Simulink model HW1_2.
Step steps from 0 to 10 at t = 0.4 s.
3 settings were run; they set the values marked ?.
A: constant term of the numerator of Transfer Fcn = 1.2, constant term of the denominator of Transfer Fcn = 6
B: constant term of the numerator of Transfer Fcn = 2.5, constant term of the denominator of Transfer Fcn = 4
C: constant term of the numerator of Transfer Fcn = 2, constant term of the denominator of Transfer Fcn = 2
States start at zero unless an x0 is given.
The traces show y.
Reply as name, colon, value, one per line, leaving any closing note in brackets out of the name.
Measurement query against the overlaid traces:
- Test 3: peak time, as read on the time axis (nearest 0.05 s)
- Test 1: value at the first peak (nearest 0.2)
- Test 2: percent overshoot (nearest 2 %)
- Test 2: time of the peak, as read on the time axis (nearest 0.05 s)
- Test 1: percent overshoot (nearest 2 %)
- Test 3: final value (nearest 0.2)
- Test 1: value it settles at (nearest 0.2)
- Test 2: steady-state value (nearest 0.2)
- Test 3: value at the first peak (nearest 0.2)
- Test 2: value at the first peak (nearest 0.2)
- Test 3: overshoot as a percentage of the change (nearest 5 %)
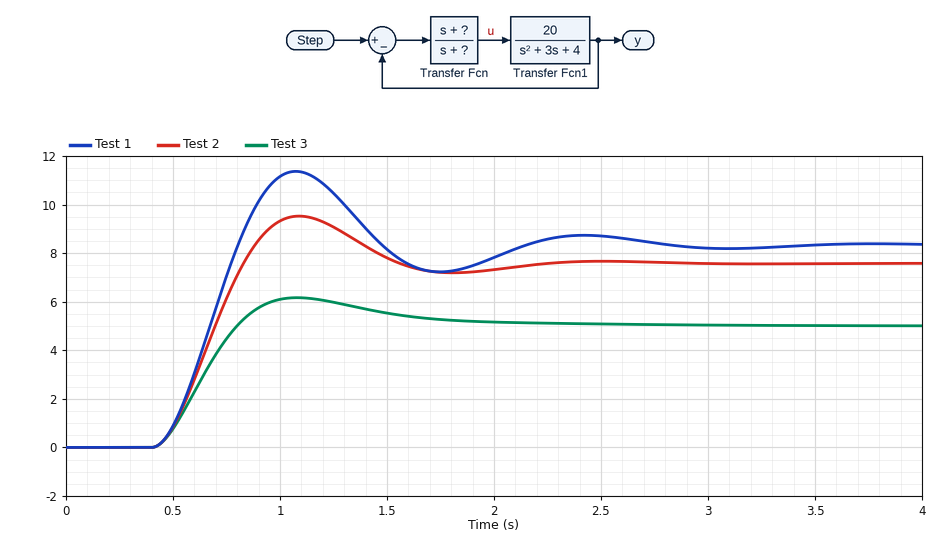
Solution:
Test 3: peak time, as read on the time axis: 1.10 s
Test 1: value at the first peak: 11.4
Test 2: percent overshoot: 26 %
Test 2: time of the peak, as read on the time axis: 1.10 s
Test 1: percent overshoot: 36 %
Test 3: final value: 5.0
Test 1: value it settles at: 8.4
Test 2: steady-state value: 7.6
Test 3: value at the first peak: 6.2
Test 2: value at the first peak: 9.6
Test 3: overshoot as a percentage of the change: 25 %
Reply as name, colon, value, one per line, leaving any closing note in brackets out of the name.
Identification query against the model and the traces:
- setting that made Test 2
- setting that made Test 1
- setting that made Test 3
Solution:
setting that made Test 2: B
setting that made Test 1: C
setting that made Test 3: A
